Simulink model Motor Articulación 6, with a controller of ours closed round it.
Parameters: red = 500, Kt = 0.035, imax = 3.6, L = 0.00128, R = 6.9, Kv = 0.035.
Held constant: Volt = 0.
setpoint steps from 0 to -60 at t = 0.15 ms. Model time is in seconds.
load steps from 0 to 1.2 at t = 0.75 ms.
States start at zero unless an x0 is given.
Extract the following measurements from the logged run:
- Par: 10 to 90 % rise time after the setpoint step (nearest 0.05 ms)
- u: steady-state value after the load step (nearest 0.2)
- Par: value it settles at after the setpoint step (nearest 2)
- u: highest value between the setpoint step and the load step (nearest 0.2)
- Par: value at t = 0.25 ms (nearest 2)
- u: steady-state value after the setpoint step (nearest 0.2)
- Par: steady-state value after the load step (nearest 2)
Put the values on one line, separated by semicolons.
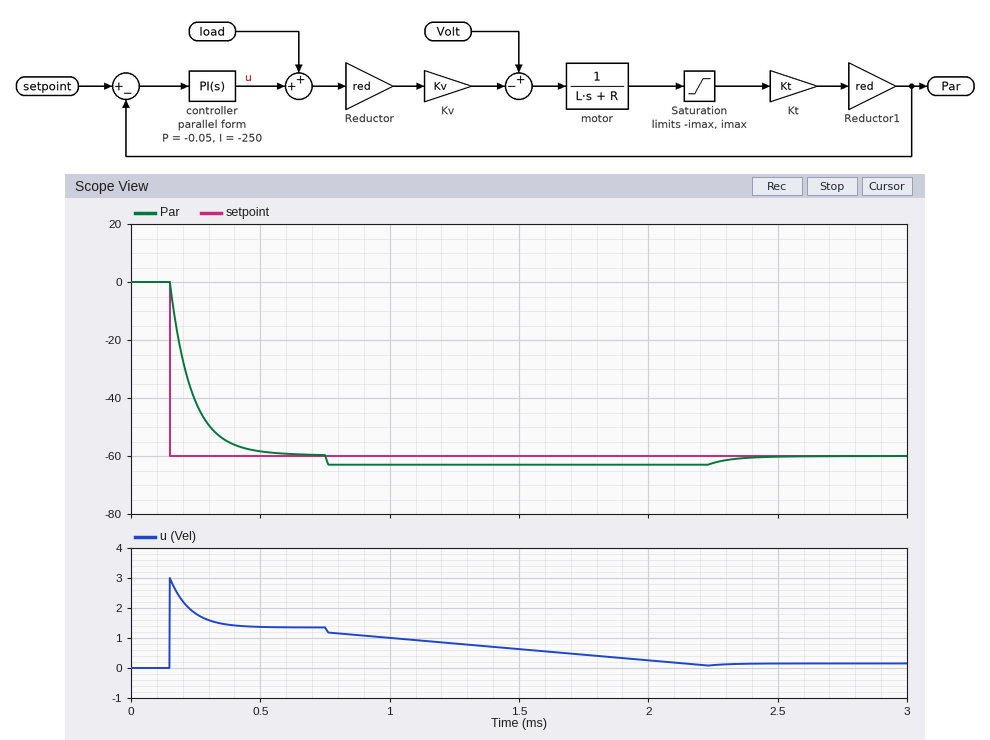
0.20 ms; 0.2; -60; 3.0; -42; 1.4; -60
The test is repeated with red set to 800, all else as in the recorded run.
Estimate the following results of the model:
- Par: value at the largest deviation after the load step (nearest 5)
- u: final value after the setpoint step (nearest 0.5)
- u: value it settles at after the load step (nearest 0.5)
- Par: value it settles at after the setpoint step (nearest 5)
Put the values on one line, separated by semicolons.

-75; 0.5; -0.5; -60
